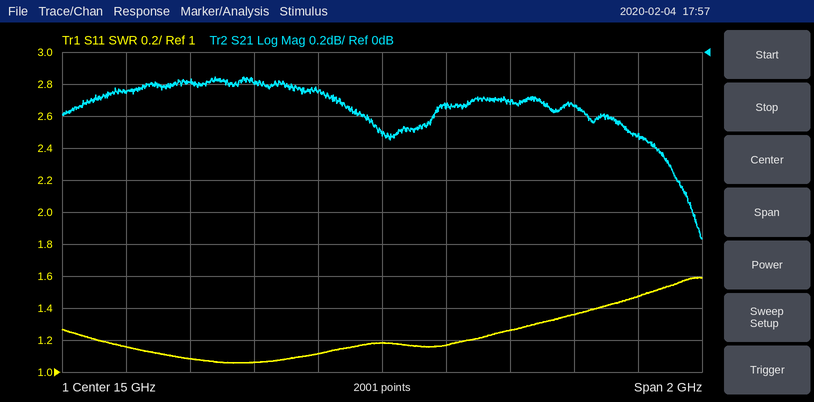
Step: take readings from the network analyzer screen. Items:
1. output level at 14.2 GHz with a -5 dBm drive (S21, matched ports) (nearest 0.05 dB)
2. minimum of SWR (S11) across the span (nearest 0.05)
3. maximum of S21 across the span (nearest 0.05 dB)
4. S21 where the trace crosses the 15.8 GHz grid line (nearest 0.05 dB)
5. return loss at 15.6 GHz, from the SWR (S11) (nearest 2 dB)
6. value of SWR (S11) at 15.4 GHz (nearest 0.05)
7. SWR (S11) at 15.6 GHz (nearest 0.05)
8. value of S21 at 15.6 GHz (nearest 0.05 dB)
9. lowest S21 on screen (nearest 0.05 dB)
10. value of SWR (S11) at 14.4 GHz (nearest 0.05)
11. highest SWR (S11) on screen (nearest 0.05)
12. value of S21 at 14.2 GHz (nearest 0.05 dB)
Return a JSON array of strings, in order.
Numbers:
["-5.25 dBm", "1.05", "-0.15 dB", "-0.50 dB", "16 dB", "1.25", "1.35", "-0.35 dB", "-1.15 dB", "1.10", "1.60", "-0.25 dB"]
